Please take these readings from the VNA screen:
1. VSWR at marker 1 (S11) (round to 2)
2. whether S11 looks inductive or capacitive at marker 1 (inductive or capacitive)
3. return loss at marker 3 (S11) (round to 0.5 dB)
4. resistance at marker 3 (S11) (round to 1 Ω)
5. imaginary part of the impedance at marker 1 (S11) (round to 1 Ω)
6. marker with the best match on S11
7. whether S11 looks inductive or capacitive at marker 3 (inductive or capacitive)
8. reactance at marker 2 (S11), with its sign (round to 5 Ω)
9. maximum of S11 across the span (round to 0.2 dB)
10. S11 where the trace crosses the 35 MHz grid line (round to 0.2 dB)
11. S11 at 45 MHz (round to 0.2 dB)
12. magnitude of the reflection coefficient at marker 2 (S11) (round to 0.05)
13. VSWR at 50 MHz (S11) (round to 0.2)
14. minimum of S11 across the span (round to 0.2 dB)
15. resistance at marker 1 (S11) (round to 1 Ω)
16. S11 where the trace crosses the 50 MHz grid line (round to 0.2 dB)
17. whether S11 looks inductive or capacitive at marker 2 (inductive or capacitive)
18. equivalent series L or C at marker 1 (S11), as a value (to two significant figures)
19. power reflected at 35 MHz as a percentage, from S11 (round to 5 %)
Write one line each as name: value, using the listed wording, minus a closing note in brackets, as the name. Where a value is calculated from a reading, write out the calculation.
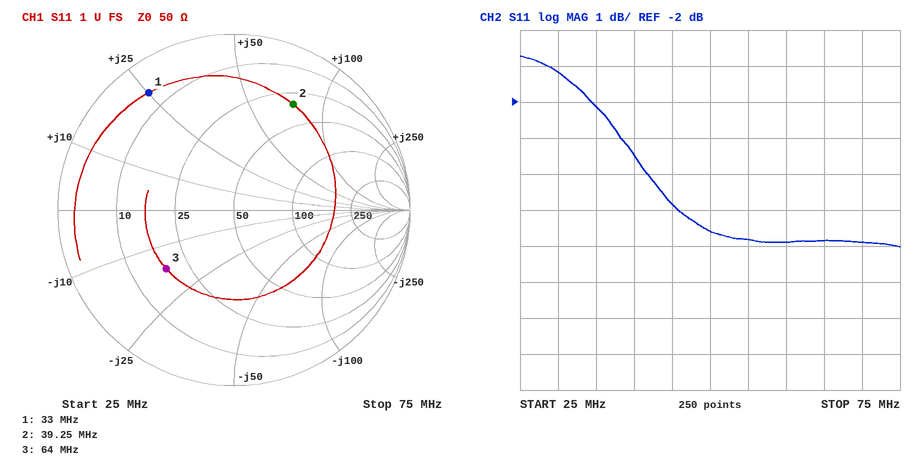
VSWR at marker 1 (S11): 10
whether S11 looks inductive or capacitive at marker 1: inductive
return loss at marker 3 (S11): 6.0 dB
resistance at marker 3 (S11): 18 Ω
imaginary part of the impedance at marker 1 (S11): +25 Ω
marker with the best match on S11: marker 3
whether S11 looks inductive or capacitive at marker 3: capacitive
reactance at marker 2 (S11), with its sign: +75 Ω
maximum of S11 across the span: -0.8 dB
S11 where the trace crosses the 35 MHz grid line: -2.2 dB
S11 at 45 MHz: -4.8 dB
magnitude of the reflection coefficient at marker 2 (S11): 0.70
VSWR at 50 MHz (S11): |Γ| = 10^(-5.6/20) = 0.5248; VSWR = (1 + 0.5248)/(1 − 0.5248) ≈ 3.2
minimum of S11 across the span: -6.0 dB
resistance at marker 1 (S11): 6 Ω
S11 where the trace crosses the 50 MHz grid line: -5.6 dB
whether S11 looks inductive or capacitive at marker 2: inductive
equivalent series L or C at marker 1 (S11), as a value: L = 25 Ω/(2π × 33 MHz) ≈ 121 nH, so 120 nH to two significant figures
power reflected at 35 MHz as a percentage, from S11: 10^(-2.2/10) ≈ 60 %
